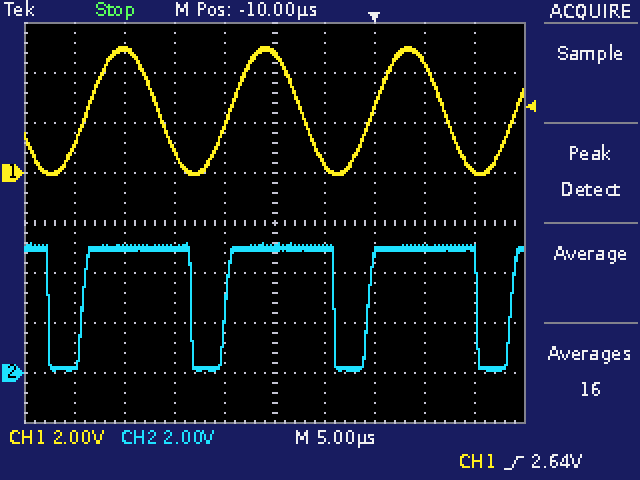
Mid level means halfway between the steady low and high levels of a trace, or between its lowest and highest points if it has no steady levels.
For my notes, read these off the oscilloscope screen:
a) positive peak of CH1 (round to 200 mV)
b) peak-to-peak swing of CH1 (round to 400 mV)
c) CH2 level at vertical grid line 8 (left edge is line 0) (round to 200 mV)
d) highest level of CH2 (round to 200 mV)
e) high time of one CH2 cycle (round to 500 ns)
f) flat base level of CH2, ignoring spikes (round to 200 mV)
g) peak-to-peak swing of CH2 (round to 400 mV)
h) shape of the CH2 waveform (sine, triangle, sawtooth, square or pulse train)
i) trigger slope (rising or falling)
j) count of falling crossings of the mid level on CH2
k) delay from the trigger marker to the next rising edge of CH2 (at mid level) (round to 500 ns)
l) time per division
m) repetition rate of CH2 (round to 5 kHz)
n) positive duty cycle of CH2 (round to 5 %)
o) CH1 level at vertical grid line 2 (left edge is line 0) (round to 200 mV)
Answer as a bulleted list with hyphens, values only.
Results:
- 5.0 V
- 5.2 V
- 5.0 V
- 5.2 V
- 11.0 µs
- 200 mV
- 5.2 V
- pulse train
- rising
- 4
- 13.5 µs
- 5 µs
- 70 kHz
- 75 %
- 5.0 V
